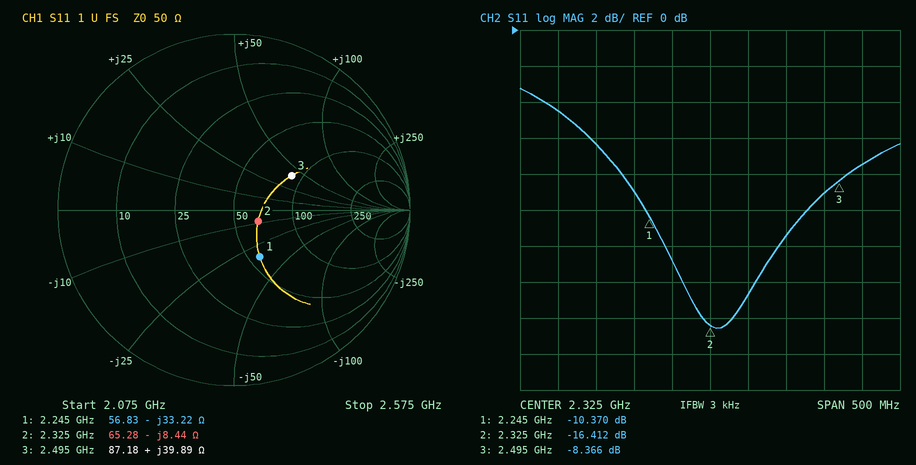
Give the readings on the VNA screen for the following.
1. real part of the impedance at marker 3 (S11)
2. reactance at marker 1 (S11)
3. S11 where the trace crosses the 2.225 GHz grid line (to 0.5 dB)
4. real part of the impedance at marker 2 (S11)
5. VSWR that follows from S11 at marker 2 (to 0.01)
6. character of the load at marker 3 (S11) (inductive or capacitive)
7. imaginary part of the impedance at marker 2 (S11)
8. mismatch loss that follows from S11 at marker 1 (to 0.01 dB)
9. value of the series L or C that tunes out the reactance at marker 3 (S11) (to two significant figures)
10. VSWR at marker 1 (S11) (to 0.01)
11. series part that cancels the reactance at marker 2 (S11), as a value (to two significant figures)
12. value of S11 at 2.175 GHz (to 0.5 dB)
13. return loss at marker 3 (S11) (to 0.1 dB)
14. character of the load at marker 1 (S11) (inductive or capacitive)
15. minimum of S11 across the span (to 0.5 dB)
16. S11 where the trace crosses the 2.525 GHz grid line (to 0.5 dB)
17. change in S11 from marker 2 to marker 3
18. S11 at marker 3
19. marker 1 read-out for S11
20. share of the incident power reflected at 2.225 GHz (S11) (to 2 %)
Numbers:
87.18 Ω
-33.22 Ω
-9.0 dB
65.28 Ω
1.36
inductive
-8.44 Ω
0.42 dB
1.6 pF
1.87
580 pH
-6.5 dB
8.4 dB
capacitive
-16.5 dB
-7.5 dB
8.046 dB
-8.366 dB
-10.370 dB
12 %
